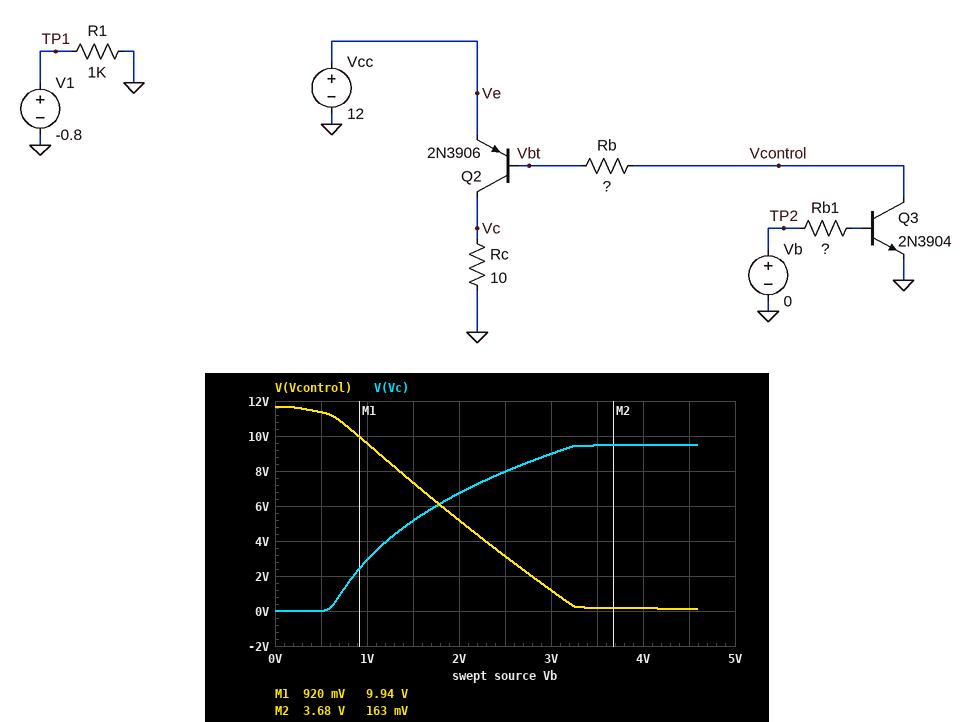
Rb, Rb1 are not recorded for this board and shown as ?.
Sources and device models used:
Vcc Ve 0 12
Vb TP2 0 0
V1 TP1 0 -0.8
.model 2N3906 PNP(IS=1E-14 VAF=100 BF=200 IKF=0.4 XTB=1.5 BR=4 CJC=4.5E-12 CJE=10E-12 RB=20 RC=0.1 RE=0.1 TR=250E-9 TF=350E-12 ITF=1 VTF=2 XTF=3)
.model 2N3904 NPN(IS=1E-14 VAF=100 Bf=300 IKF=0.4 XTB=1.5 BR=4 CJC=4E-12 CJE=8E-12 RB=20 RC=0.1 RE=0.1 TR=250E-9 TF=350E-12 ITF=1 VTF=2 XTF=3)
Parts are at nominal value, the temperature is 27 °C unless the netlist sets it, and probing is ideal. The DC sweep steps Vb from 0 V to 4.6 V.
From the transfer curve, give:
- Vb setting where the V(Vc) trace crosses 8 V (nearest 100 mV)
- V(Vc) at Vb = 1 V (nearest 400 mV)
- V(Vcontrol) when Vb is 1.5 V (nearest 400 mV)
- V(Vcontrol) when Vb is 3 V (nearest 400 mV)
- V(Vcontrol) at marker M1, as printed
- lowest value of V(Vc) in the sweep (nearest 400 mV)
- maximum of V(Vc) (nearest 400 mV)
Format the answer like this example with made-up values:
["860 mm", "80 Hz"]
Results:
["2.5 V", "2.8 V", "7.2 V", "1.2 V", "9.94 V", "0 V", "9.6 V"]
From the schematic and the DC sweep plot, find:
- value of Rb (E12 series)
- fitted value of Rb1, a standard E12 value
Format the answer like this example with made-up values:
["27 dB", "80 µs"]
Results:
["680 Ω", "47 kΩ"]
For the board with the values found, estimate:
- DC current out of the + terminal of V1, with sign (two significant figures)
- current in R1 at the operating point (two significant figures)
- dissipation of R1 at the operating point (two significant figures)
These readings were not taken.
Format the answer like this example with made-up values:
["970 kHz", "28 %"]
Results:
["-800 µA", "800 µA", "640 µW"]
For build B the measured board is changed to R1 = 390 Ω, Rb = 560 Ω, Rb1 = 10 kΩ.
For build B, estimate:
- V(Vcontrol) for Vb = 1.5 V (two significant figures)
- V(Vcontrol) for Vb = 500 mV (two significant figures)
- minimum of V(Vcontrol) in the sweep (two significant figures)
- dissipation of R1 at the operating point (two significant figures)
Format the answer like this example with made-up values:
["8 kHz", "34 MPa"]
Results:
["160 mV", "11 V", "77 mV", "1.6 mW"]
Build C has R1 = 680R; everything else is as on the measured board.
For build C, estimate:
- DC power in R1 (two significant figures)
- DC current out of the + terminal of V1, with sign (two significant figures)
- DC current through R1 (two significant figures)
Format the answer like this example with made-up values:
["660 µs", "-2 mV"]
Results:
["940 µW", "-1.2 mA", "1.2 mA"]
